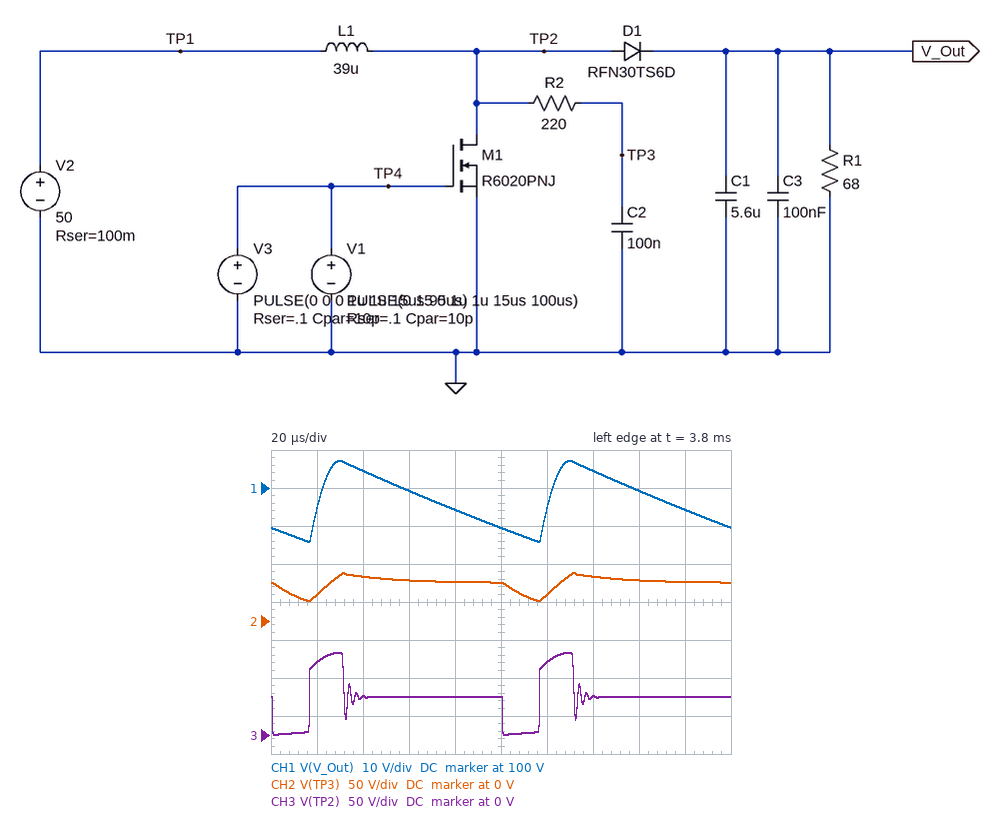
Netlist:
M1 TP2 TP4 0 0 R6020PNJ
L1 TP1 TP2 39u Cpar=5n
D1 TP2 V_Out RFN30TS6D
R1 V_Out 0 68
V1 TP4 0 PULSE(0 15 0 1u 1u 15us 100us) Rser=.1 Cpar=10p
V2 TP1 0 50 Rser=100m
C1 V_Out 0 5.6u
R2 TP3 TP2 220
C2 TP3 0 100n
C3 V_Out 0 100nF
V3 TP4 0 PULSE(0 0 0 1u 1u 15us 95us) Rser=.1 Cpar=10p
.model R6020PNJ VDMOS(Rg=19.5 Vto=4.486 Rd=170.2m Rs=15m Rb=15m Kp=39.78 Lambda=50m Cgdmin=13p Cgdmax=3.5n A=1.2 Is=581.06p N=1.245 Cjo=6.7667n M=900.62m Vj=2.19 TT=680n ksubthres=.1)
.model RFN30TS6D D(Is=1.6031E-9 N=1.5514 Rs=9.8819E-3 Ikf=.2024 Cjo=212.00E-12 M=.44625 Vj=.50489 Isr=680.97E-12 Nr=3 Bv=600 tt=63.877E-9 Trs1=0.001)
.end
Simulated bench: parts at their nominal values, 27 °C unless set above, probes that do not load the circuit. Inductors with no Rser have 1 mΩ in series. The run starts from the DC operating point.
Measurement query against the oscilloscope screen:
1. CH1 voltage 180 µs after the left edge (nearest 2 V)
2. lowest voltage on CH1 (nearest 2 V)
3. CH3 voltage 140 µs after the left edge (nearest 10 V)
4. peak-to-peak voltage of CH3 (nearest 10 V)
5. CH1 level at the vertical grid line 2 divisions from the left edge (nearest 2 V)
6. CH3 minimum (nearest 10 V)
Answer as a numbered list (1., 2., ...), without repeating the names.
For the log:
1. 94 V
2. 86 V
3. 50 V
4. 110 V
5. 104 V
6. 0 V
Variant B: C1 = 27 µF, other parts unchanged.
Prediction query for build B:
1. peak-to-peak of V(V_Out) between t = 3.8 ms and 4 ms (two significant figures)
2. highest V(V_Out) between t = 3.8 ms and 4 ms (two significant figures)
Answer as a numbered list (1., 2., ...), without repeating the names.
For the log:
1. 4.5 V
2. 99 V
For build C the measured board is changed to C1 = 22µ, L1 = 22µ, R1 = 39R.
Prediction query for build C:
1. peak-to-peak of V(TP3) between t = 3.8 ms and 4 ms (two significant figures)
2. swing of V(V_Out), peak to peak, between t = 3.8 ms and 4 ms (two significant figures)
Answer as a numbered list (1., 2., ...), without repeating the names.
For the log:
1. 35 V
2. 9.3 V
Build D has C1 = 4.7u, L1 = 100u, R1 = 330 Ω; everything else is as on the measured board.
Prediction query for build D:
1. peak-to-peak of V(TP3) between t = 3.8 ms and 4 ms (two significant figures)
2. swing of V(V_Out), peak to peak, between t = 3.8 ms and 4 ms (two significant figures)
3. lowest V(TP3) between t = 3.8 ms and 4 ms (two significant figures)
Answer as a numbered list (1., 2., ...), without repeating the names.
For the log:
1. 39 V
2. 7.0 V
3. 25 V
